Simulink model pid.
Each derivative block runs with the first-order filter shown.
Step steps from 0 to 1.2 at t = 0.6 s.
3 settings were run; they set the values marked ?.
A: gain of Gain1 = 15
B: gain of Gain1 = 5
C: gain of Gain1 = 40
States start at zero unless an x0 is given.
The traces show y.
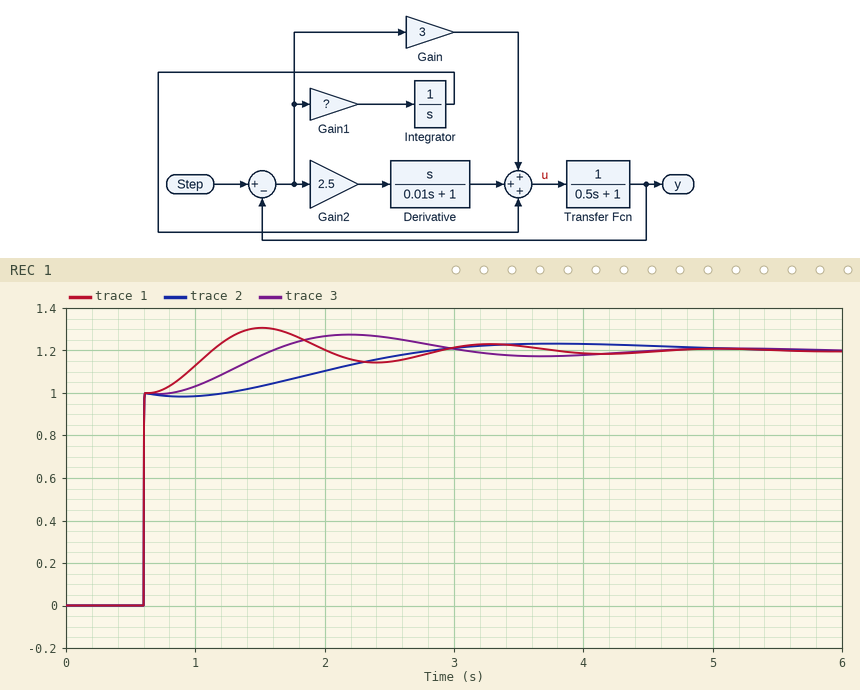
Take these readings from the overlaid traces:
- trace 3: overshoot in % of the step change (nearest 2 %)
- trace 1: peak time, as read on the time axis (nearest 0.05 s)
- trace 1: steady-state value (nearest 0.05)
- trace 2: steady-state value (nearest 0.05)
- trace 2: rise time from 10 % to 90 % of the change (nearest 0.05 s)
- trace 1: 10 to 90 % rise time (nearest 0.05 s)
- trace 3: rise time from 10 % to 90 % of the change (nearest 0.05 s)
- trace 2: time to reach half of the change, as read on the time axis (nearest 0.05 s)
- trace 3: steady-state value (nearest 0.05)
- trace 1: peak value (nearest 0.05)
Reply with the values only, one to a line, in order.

6 %
1.50 s
1.20
1.20
1.25 s
0.30 s
0.60 s
0.60 s
1.20
1.30
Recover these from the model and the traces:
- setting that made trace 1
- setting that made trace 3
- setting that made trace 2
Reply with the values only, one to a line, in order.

C
A
B
